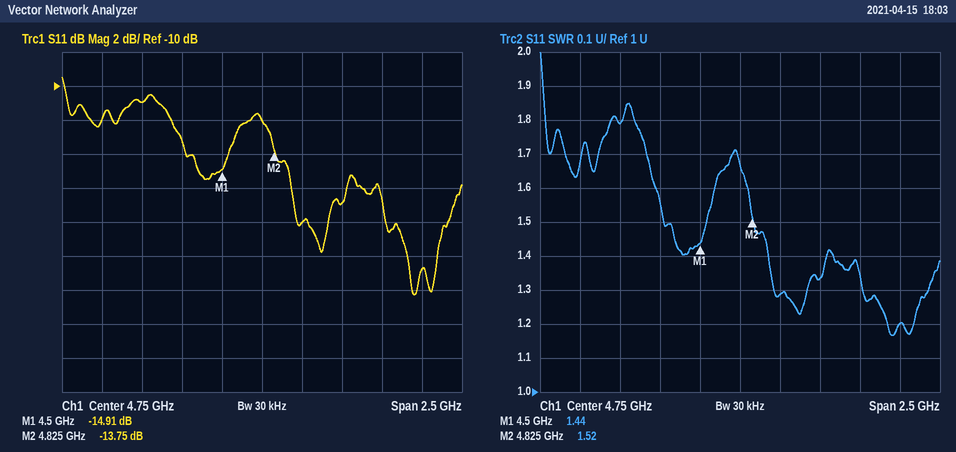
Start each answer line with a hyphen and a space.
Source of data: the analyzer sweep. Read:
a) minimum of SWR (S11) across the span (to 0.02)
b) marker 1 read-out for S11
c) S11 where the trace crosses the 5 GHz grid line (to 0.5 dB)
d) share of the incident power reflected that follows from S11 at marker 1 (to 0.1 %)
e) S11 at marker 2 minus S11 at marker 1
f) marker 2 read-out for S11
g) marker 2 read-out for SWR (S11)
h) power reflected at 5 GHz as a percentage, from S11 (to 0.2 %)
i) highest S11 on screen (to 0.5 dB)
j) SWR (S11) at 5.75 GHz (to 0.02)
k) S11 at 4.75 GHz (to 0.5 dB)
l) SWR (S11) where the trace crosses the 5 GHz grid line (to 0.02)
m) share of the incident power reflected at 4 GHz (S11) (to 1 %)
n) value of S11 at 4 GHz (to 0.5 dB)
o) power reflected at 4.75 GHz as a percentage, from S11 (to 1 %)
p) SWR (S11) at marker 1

- 1.16
- -14.91 dB
- -18.0 dB
- 3.2 %
- 1.16 dB
- -13.75 dB
- 1.52
- 1.6 %
- -9.5 dB
- 1.20
- -12.0 dB
- 1.28
- 8 %
- -11.0 dB
- 6 %
- 1.44
